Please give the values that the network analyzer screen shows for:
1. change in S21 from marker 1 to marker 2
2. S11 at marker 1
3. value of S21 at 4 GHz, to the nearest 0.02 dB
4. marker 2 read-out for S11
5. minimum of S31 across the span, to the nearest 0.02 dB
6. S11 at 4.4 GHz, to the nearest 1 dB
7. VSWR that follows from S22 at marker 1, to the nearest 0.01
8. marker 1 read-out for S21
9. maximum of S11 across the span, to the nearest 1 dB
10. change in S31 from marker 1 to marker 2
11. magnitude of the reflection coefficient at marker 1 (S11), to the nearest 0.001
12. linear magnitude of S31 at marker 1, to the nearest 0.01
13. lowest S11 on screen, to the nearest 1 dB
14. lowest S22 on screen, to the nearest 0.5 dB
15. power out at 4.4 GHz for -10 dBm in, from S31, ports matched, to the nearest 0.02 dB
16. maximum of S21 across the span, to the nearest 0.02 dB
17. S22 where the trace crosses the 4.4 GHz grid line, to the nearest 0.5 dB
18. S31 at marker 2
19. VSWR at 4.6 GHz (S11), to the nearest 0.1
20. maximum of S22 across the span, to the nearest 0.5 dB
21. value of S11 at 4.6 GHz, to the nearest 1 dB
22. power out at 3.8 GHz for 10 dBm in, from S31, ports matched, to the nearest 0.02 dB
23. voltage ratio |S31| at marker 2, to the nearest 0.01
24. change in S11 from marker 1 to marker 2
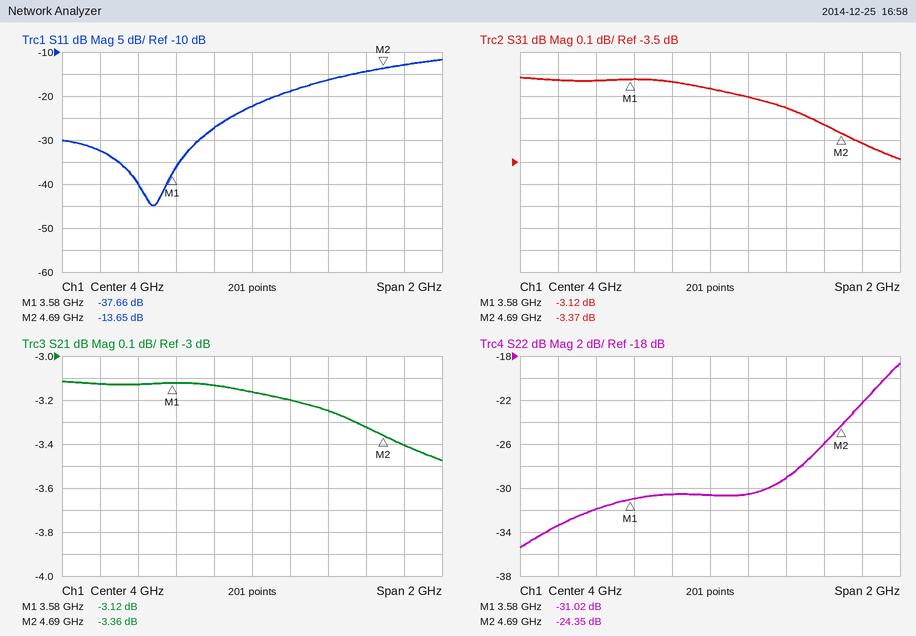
-0.24 dB
-37.66 dB
-3.16 dB
-13.65 dB
-3.48 dB
-16 dB
1.06
-3.12 dB
-12 dB
-0.25 dB
0.013
0.70
-45 dB
-35.5 dB
-13.26 dBm
-3.12 dB
-29.0 dB
-3.37 dB
1.5
-18.5 dB
-14 dB
6.86 dBm
0.68
24.01 dB
